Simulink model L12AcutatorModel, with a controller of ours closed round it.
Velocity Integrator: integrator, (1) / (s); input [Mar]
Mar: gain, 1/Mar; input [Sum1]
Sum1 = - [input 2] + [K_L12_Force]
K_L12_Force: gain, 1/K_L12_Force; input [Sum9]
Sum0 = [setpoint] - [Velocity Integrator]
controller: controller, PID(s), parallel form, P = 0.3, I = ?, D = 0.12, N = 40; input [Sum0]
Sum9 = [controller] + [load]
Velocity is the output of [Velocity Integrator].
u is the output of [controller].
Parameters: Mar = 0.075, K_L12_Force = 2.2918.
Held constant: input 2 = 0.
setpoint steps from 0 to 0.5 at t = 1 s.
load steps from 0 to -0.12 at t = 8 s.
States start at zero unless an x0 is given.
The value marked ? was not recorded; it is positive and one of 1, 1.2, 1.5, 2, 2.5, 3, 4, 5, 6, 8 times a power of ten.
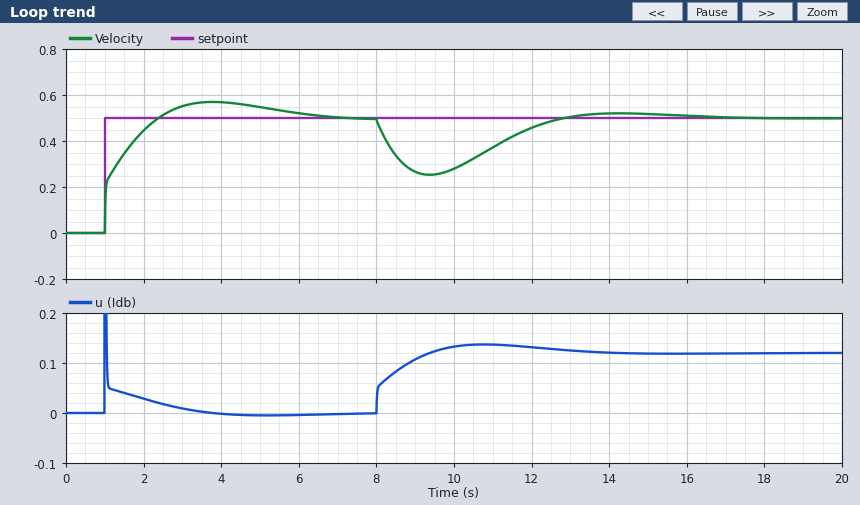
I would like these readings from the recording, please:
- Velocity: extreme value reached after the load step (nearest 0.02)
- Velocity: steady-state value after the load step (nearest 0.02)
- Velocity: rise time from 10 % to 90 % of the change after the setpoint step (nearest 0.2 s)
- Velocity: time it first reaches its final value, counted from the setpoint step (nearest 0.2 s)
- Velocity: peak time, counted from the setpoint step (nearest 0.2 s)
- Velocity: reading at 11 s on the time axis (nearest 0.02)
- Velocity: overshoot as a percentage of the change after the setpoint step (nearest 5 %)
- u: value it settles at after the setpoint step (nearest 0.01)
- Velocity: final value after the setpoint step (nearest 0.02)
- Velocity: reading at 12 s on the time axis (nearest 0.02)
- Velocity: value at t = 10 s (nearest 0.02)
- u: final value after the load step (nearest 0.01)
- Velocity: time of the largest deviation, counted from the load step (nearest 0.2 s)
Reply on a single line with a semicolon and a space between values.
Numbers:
0.26; 0.50; 1.0 s; 1.4 s; 2.8 s; 0.38; 15 %; 0.00; 0.50; 0.46; 0.28; 0.12; 1.4 s
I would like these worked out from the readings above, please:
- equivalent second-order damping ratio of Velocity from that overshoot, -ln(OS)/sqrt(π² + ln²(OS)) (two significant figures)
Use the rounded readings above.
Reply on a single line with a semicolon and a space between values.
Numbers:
0.52
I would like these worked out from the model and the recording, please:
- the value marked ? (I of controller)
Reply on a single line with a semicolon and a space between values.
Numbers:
0.2
